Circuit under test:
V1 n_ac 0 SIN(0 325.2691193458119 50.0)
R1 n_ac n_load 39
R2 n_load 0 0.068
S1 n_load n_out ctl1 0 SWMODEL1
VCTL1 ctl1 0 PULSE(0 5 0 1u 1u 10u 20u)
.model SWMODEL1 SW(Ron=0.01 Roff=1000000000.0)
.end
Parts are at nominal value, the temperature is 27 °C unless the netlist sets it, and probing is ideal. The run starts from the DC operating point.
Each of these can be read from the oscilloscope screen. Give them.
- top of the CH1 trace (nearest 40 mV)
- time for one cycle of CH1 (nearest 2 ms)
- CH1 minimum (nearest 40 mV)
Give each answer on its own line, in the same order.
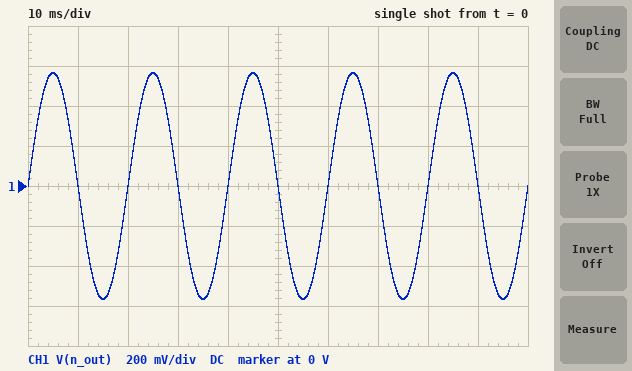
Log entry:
560 mV
20 ms
-560 mV
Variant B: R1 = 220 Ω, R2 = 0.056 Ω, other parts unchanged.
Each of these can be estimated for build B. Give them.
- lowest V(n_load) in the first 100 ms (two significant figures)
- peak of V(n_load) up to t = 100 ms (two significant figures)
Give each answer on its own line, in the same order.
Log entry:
-83 mV
83 mV
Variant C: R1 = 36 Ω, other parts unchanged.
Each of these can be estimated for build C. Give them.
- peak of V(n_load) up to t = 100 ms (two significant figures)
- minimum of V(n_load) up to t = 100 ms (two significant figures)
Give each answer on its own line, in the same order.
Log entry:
610 mV
-610 mV
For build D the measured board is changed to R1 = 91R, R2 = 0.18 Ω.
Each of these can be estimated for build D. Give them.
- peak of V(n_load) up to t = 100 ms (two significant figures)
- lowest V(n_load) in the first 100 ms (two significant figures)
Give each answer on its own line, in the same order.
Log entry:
640 mV
-640 mV
